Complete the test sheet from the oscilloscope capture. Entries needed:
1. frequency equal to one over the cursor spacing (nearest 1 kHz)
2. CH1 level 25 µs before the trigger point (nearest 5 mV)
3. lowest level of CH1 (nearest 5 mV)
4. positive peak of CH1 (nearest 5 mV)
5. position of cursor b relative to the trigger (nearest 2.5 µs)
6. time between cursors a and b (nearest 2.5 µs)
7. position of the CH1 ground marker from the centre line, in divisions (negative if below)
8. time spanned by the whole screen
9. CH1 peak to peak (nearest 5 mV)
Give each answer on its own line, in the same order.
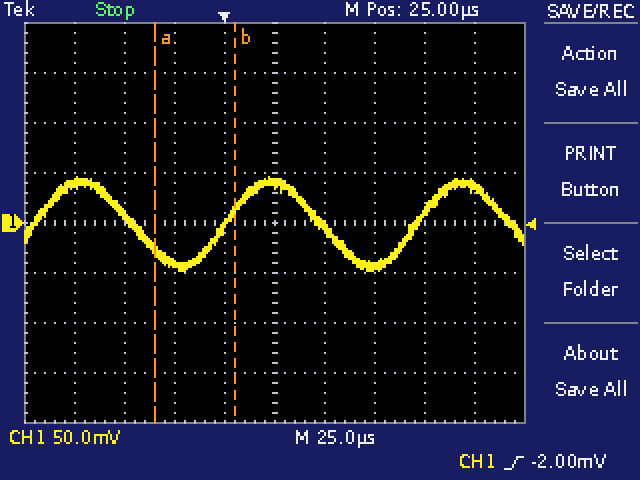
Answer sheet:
25 kHz
-40 mV
-50 mV
45 mV
+5.0 µs
40.0 µs
0.0 div
250 µs
95 mV
